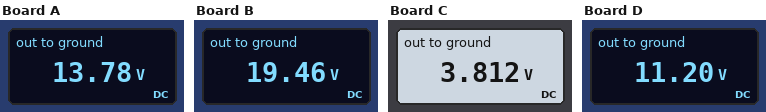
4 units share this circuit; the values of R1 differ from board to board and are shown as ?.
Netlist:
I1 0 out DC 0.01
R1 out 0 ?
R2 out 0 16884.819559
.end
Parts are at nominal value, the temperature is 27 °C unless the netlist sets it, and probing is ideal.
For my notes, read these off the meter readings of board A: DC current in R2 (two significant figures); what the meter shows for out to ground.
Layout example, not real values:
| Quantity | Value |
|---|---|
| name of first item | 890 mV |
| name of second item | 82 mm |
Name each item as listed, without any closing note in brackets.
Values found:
| Quantity | Value |
|---|---|
| DC current in R2 | 820 µA |
| what the meter shows for out to ground | 13.78 V |
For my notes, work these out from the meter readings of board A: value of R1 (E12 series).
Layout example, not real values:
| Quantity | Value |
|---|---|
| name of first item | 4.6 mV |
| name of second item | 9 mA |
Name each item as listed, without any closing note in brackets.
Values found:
| Quantity | Value |
|---|---|
| value of R1 | 1.5 kΩ |
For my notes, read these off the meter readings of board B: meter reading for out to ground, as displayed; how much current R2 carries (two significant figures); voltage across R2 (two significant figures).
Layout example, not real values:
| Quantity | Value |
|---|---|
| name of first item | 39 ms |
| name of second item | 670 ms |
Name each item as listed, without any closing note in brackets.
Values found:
| Quantity | Value |
|---|---|
| meter reading for out to ground, as displayed | 19.46 V |
| how much current R2 carries | 1.2 mA |
| voltage across R2 | 19 V |
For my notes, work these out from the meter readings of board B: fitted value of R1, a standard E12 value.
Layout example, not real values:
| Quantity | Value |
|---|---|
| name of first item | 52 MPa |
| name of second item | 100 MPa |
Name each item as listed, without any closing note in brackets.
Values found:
| Quantity | Value |
|---|---|
| fitted value of R1, a standard E12 value | 2.2 kΩ |
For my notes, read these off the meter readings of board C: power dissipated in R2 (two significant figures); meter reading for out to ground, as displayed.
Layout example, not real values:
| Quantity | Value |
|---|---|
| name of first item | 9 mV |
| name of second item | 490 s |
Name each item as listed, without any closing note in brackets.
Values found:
| Quantity | Value |
|---|---|
| power dissipated in R2 | 860 µW |
| meter reading for out to ground, as displayed | 3.812 V |
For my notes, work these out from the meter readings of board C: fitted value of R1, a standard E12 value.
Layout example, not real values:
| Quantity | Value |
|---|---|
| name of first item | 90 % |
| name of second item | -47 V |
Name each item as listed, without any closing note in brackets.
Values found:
| Quantity | Value |
|---|---|
| fitted value of R1, a standard E12 value | 390 Ω |
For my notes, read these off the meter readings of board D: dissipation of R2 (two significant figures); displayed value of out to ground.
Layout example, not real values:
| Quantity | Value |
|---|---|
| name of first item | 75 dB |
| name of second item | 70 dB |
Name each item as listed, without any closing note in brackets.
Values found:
| Quantity | Value |
|---|---|
| dissipation of R2 | 7.4 mW |
| displayed value of out to ground | 11.20 V |
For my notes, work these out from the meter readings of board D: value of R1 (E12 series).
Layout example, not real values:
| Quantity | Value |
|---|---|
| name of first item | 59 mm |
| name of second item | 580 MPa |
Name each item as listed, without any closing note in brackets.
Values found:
| Quantity | Value |
|---|---|
| value of R1 | 1.2 kΩ |
